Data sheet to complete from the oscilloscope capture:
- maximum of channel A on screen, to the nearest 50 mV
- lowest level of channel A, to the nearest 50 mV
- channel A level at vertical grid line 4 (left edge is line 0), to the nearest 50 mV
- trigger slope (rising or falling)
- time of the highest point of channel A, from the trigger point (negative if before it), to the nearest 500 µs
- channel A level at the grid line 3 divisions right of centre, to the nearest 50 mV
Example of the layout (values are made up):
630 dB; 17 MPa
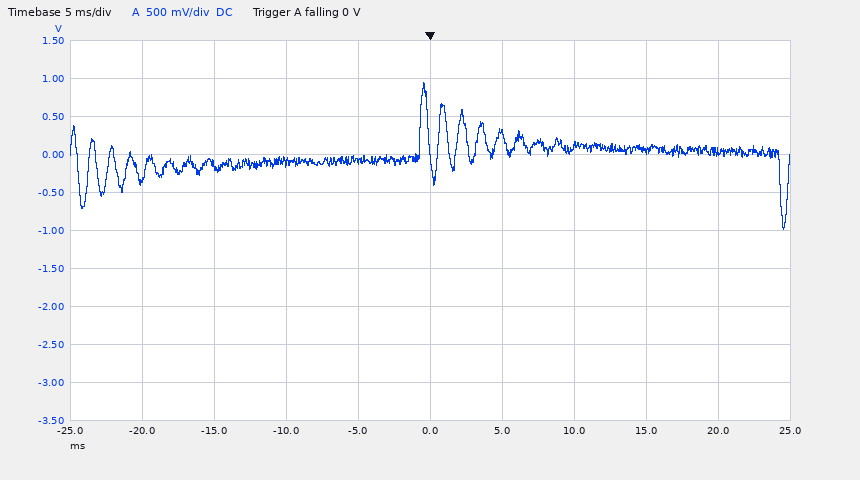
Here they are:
950 mV; -1.00 V; -100 mV; falling; -500 µs; 50 mV
